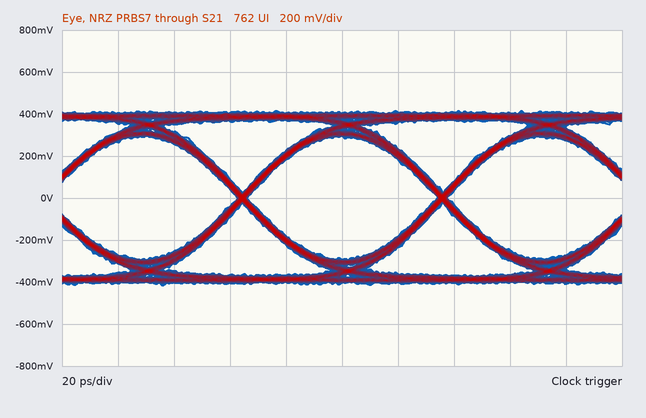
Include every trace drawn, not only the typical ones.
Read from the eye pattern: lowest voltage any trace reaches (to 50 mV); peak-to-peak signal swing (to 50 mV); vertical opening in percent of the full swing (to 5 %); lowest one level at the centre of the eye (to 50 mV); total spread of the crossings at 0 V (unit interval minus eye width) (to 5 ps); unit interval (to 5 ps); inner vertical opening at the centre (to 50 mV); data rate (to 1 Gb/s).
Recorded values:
-400 mV
850 mV
70 %
300 mV
5 ps
70 ps
600 mV
14 Gb/s
